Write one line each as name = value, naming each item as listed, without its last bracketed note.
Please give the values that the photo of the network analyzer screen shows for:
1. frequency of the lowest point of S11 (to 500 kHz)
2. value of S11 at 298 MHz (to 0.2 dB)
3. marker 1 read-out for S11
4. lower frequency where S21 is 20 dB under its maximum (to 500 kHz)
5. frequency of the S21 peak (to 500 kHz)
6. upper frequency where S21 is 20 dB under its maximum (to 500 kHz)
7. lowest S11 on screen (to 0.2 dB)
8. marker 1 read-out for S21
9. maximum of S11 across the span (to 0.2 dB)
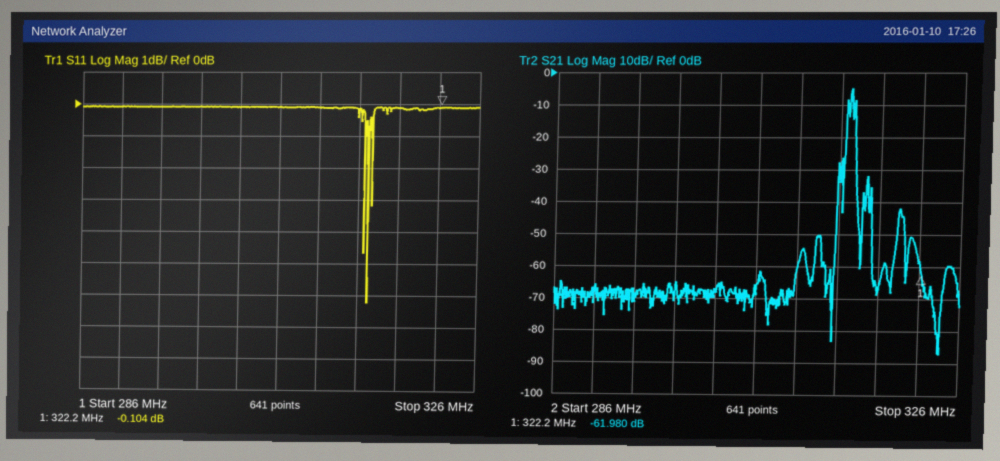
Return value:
frequency of the lowest point of S11 = 315.0 MHz
value of S11 at 298 MHz = 0.0 dB
marker 1 read-out for S11 = -0.104 dB
lower frequency where S21 is 20 dB under its maximum = 314.5 MHz
frequency of the S21 peak = 315.0 MHz
upper frequency where S21 is 20 dB under its maximum = 315.5 MHz
lowest S11 on screen = -6.2 dB
marker 1 read-out for S21 = -61.980 dB
maximum of S11 across the span = 0.0 dB
